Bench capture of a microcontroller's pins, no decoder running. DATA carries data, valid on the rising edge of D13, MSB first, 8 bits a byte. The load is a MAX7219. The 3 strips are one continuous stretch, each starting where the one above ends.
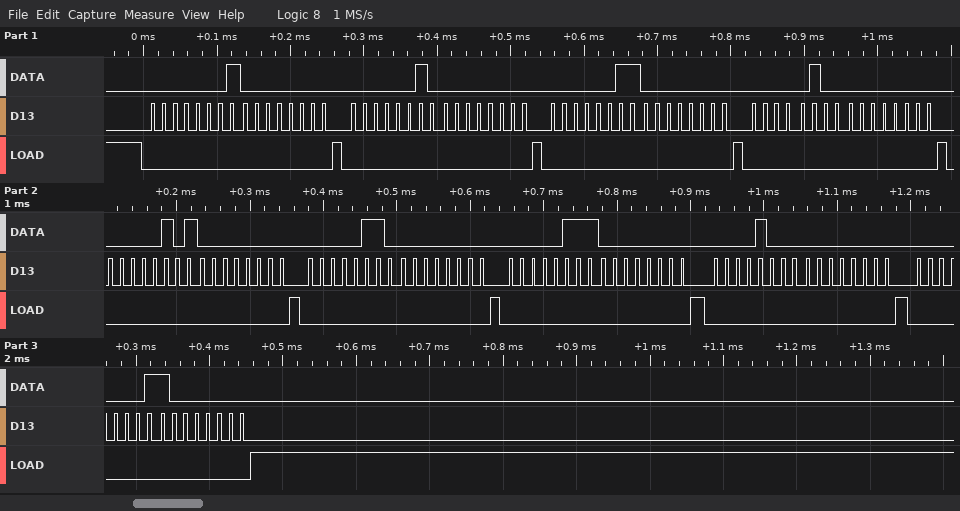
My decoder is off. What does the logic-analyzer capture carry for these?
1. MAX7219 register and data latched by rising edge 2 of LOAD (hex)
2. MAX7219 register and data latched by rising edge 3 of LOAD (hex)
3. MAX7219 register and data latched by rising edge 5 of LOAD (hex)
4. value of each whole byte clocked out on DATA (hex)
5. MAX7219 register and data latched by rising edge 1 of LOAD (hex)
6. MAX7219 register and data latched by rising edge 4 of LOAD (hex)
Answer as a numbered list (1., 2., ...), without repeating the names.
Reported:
1. register 0x2, data 0x00
2. register 0x3, data 0x00
3. register 0x5, data 0x00
4. 0x01 0x00 0x02 0x00 0x03 0x00 0x04 0x00 0x05 0x00 0x06 0x00 0x07 0x00 0x08 0x00 0x01 0x80
5. register 0x1, data 0x00
6. register 0x4, data 0x00
